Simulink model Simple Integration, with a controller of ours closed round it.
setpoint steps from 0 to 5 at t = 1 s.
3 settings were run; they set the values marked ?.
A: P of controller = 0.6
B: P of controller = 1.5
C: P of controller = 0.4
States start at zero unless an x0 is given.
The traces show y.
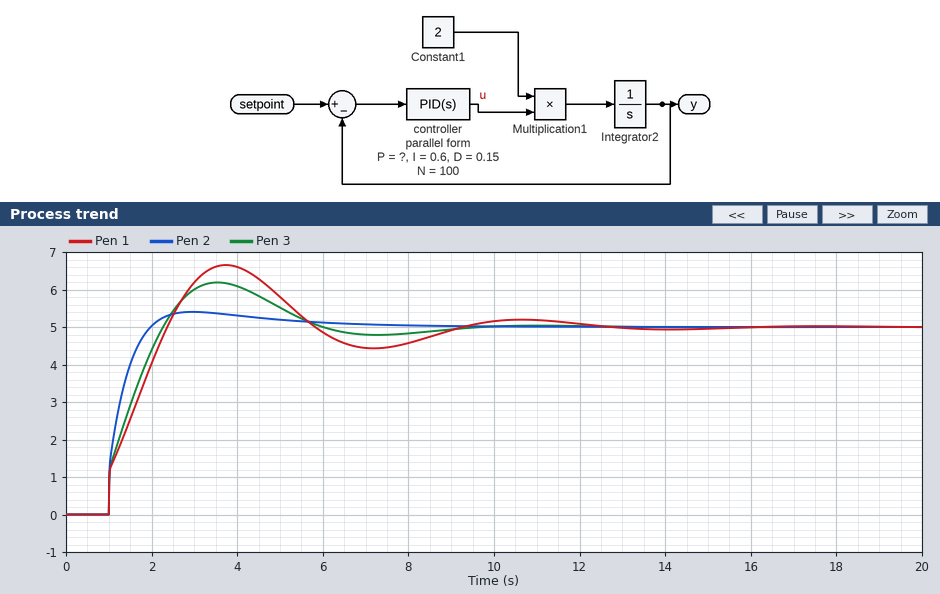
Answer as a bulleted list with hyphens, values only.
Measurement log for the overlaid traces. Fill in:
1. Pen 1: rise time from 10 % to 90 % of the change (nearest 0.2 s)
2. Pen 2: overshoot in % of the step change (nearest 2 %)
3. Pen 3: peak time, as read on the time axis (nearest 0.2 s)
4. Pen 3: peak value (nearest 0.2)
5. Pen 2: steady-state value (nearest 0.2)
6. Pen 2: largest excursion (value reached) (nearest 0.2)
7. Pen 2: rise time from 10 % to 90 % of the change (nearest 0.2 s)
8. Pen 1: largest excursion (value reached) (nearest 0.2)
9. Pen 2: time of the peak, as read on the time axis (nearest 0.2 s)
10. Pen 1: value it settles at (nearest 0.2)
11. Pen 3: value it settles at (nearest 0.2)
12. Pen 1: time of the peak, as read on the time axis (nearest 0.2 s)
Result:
- 1.2 s
- 8 %
- 3.6 s
- 6.2
- 5.0
- 5.4
- 0.6 s
- 6.6
- 3.0 s
- 5.0
- 5.0
- 3.8 s
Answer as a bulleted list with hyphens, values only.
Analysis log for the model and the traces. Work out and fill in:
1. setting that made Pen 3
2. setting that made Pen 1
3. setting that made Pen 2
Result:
- A
- C
- B
